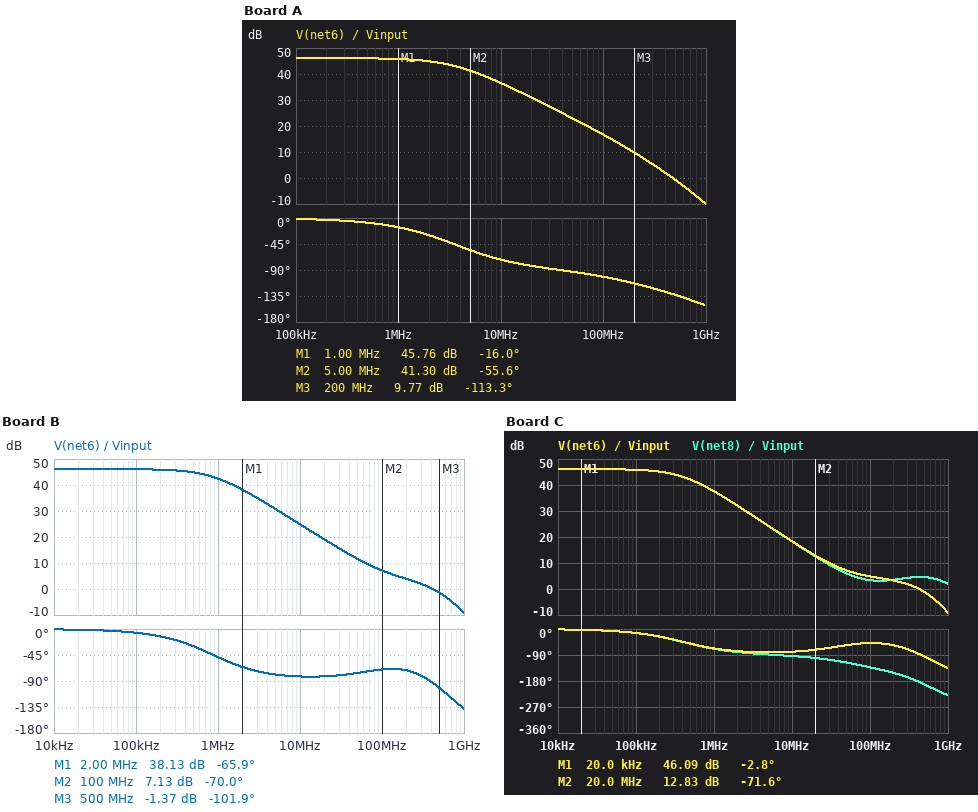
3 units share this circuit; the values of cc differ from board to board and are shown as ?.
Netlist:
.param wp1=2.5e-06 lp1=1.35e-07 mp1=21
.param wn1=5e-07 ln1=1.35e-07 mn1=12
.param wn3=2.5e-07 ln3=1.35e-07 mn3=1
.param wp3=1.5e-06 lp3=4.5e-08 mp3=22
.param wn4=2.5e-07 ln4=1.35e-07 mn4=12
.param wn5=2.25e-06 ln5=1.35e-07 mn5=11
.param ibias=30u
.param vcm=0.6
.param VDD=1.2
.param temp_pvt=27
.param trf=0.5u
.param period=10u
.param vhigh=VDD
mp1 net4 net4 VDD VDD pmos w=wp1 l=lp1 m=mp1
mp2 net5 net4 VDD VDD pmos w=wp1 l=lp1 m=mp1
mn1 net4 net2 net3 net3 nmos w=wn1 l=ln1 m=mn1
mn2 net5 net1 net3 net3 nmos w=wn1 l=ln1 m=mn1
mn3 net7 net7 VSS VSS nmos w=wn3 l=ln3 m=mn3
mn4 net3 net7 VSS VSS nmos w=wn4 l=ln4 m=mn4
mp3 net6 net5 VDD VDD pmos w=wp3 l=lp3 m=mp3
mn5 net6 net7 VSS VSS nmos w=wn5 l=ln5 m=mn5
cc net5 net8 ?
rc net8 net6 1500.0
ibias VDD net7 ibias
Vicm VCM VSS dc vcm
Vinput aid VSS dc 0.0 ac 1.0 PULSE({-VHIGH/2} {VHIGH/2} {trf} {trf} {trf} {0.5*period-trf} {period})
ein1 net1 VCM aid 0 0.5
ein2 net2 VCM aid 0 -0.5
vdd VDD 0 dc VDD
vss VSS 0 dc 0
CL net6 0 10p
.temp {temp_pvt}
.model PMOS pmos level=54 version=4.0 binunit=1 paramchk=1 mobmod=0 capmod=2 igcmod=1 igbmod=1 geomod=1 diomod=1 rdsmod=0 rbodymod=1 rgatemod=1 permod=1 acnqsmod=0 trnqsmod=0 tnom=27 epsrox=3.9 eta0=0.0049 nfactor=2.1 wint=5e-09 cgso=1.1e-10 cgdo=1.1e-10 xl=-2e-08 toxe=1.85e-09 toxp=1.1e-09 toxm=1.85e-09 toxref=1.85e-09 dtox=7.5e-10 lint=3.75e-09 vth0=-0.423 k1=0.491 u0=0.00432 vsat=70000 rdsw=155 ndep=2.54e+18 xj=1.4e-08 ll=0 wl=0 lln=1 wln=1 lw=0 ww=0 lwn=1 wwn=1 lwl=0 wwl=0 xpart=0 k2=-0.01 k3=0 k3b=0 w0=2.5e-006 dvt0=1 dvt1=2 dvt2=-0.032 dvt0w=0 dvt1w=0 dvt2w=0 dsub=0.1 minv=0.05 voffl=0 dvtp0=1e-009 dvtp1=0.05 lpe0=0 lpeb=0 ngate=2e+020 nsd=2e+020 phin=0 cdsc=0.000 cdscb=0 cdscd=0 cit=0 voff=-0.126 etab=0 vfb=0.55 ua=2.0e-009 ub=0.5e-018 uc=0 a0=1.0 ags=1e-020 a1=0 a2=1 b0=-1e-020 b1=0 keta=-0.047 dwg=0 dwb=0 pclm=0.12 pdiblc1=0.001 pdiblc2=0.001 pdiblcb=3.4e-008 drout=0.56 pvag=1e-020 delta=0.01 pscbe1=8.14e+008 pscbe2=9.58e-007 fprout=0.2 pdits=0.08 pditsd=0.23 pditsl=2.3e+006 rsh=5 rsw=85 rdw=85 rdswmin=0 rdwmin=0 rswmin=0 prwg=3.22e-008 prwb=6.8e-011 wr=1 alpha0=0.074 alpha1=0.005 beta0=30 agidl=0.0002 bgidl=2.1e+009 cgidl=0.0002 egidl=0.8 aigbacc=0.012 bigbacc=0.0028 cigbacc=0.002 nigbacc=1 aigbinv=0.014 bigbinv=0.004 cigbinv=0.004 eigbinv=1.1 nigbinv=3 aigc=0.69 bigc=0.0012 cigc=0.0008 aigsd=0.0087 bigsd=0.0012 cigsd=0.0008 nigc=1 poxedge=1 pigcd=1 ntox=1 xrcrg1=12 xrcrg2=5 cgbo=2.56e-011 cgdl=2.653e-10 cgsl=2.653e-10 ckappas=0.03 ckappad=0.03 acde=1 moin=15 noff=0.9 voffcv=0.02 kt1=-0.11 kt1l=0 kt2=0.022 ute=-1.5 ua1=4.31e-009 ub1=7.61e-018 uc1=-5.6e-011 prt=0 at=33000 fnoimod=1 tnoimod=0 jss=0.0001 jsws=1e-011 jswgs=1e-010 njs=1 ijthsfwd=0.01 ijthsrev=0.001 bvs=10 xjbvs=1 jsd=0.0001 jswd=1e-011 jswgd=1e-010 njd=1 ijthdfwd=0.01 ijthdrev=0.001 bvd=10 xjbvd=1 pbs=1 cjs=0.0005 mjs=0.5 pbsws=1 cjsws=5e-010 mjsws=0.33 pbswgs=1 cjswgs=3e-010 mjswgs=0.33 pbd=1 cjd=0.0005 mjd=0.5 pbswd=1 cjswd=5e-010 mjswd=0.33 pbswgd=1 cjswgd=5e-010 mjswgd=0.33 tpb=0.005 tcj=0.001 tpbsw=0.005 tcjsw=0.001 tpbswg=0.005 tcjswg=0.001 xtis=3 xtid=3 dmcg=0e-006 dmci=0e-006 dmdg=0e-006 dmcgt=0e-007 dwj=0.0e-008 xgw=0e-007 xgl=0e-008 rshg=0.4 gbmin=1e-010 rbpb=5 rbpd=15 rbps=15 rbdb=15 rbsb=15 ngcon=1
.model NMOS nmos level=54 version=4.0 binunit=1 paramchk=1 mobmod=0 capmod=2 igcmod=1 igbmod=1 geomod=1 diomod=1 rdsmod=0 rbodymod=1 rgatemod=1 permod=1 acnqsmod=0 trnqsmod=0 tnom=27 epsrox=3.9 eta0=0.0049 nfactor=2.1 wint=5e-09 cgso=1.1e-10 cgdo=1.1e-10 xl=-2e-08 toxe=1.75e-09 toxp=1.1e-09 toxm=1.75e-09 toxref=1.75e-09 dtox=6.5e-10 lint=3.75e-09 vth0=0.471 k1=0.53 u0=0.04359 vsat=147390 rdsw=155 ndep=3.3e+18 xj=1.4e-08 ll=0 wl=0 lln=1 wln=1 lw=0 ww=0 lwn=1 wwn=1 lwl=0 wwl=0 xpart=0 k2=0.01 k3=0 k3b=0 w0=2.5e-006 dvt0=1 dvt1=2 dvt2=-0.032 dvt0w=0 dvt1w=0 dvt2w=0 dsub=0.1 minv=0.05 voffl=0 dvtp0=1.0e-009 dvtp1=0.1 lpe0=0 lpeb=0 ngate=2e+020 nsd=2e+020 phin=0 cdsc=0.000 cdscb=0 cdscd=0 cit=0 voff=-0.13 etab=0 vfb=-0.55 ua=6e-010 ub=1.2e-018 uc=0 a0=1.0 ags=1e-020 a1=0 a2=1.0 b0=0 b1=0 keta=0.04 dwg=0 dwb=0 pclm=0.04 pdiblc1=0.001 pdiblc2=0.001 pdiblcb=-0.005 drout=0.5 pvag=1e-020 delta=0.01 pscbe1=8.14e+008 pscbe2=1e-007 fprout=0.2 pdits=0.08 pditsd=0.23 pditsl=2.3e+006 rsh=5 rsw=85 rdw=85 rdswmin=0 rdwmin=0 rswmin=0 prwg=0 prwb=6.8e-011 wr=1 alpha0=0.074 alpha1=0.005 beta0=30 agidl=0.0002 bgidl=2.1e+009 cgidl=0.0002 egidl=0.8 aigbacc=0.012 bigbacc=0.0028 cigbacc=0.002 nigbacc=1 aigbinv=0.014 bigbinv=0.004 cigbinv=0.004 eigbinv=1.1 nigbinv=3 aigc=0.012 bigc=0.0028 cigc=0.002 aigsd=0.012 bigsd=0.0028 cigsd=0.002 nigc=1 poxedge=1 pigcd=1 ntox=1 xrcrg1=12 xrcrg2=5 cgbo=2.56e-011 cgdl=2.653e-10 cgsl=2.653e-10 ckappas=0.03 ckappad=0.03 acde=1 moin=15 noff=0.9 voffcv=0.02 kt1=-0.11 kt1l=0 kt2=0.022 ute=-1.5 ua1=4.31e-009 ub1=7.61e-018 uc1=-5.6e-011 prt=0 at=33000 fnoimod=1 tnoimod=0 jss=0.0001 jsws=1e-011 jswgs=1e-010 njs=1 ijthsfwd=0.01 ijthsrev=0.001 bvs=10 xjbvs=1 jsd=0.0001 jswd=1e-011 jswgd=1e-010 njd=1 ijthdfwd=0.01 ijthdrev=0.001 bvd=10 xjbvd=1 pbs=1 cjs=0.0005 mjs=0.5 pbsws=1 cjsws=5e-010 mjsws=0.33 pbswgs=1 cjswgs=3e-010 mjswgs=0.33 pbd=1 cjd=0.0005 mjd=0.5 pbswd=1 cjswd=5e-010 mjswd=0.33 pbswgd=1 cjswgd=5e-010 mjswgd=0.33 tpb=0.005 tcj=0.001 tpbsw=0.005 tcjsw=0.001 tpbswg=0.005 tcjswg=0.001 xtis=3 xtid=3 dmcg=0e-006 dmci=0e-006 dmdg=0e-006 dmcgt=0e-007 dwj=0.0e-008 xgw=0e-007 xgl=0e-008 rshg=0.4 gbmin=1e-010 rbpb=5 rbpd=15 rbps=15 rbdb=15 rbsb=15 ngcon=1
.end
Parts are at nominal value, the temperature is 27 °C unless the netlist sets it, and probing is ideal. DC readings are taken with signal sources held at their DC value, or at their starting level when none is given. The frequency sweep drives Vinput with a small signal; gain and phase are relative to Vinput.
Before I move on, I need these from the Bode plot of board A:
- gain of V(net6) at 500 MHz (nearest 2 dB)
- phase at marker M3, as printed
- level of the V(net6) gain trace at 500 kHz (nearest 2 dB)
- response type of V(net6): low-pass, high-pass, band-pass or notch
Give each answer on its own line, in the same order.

0 dB
-113.3 deg
46 dB
low-pass
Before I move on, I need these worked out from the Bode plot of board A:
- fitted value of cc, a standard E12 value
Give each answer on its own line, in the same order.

220 fF
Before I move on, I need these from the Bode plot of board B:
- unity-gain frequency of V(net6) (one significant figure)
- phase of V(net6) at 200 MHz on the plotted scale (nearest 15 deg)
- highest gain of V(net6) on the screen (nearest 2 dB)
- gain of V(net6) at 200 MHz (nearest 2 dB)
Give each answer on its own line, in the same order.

400 MHz
-75 deg
46 dB
4 dB
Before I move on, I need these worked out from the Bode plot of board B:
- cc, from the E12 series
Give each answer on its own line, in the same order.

1 pF
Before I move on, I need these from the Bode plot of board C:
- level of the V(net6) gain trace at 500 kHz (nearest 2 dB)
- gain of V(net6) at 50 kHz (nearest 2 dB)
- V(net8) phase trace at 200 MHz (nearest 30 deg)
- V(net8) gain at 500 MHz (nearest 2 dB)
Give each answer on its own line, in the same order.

42 dB
46 dB
-150 deg
4 dB
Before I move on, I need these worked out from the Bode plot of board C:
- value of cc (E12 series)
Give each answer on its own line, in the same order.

2.2 pF
